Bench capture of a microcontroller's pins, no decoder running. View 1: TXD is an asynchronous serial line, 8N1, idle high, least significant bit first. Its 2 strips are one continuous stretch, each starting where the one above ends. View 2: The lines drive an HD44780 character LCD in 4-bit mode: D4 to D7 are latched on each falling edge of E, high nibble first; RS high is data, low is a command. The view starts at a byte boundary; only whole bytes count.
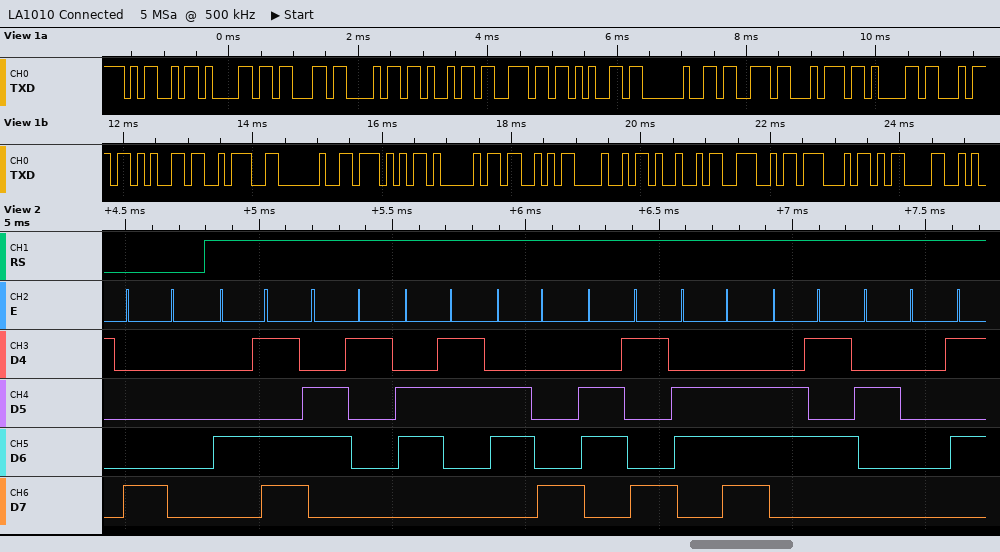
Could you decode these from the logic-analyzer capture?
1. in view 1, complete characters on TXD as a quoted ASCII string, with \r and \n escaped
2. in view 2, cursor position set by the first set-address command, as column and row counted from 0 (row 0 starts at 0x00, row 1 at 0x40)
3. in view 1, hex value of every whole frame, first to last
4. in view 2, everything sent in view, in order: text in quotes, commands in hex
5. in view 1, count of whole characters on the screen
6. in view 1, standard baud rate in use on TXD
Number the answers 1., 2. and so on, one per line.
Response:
1. "Machine state: WASHING\r"
2. column 0, row 0
3. 4D 61 63 68 69 6E 65 20 73 74 61 74 65 3A 20 57 41 53 48 49 4E 47 0D
4. 0x80 "Machine "
5. 23
6. 9600 baud
